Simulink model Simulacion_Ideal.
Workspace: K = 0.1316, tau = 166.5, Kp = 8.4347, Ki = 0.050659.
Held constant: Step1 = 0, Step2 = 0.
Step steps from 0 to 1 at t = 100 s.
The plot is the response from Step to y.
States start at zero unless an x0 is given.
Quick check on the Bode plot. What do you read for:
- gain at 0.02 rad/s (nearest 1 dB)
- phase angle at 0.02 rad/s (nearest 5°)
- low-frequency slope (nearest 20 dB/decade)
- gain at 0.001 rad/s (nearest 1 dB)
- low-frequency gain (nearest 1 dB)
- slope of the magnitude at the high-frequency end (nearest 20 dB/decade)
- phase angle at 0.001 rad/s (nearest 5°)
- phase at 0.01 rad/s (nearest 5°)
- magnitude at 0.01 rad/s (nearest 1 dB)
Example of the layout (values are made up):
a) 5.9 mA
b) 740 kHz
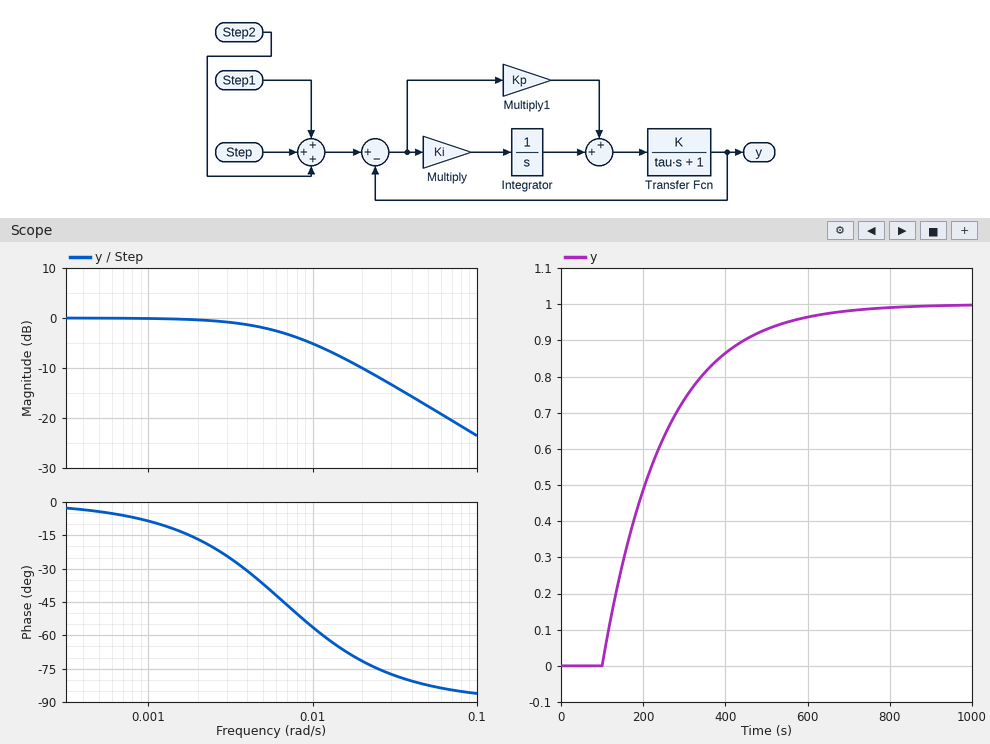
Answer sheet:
a) -10 dB
b) -70°
c) 0 dB/decade
d) 0 dB
e) 0 dB
f) -20 dB/decade
g) -10°
h) -55°
i) -5 dB
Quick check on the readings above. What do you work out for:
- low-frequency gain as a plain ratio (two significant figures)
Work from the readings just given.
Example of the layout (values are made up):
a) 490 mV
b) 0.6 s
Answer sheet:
a) 1.0
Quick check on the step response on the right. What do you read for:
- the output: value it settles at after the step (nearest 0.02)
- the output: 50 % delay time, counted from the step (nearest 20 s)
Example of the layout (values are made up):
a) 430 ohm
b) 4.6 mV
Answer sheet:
a) 1.00
b) 100 s
